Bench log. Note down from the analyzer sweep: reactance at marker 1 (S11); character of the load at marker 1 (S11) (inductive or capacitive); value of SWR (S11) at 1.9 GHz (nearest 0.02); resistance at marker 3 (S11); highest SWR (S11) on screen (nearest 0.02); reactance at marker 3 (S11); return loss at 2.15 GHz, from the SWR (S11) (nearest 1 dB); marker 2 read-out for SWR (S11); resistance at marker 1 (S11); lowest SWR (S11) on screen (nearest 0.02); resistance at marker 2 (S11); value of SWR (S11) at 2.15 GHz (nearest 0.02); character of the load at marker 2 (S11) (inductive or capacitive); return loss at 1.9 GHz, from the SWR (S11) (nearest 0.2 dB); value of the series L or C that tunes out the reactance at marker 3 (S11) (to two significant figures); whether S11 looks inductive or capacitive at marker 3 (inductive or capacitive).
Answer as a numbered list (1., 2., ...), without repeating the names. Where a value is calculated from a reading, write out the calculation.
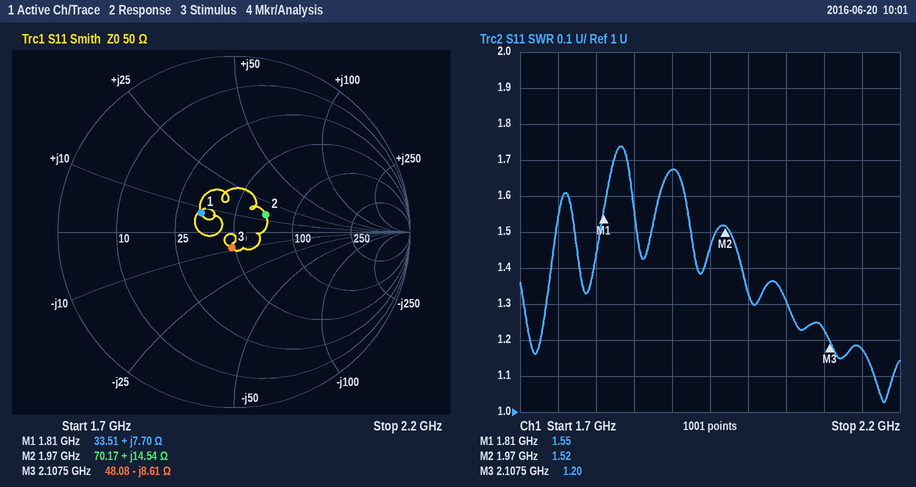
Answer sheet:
1. +7.70 Ω
2. inductive
3. 1.68
4. 48.08 Ω
5. 1.74
6. -8.61 Ω
7. −20 log10((1.18 − 1)/(1.18 + 1)) ≈ 22 dB
8. 1.52
9. 33.51 Ω
10. 1.02
11. 70.17 Ω
12. 1.18
13. inductive
14. −20 log10((1.68 − 1)/(1.68 + 1)) ≈ 11.9 dB, so 12.0 dB to the nearest 0.2 dB
15. L = 8.61 Ω/(2π × 2.1075 GHz) ≈ 650 pH
16. capacitive
